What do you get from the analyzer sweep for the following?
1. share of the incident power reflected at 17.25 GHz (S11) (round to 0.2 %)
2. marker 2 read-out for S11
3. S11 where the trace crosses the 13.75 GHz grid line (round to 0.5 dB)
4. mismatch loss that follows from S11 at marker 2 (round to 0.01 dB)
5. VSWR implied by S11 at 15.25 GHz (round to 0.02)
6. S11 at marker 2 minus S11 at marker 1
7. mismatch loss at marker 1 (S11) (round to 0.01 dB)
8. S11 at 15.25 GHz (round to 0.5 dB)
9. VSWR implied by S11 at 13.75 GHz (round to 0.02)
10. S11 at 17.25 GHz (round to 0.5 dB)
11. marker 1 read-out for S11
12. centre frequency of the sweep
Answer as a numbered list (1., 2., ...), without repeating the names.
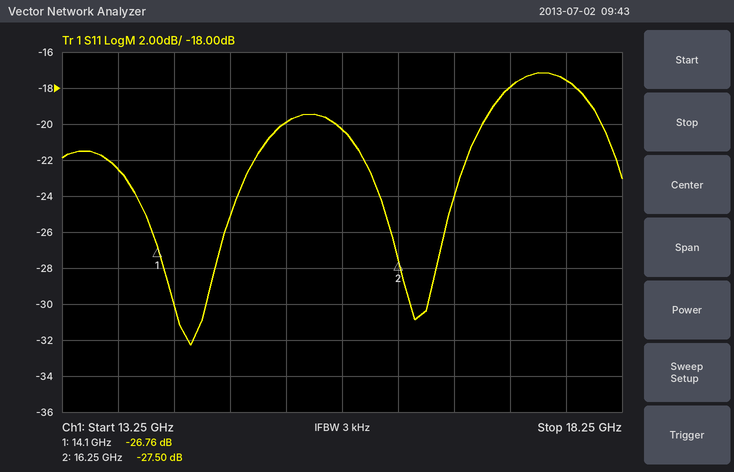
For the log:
1. 1.6 %
2. -27.50 dB
3. -22.5 dB
4. 0.01 dB
5. 1.22
6. -0.74 dB
7. 0.01 dB
8. -20.0 dB
9. 1.16
10. -18.0 dB
11. -26.76 dB
12. 15.75 GHz
